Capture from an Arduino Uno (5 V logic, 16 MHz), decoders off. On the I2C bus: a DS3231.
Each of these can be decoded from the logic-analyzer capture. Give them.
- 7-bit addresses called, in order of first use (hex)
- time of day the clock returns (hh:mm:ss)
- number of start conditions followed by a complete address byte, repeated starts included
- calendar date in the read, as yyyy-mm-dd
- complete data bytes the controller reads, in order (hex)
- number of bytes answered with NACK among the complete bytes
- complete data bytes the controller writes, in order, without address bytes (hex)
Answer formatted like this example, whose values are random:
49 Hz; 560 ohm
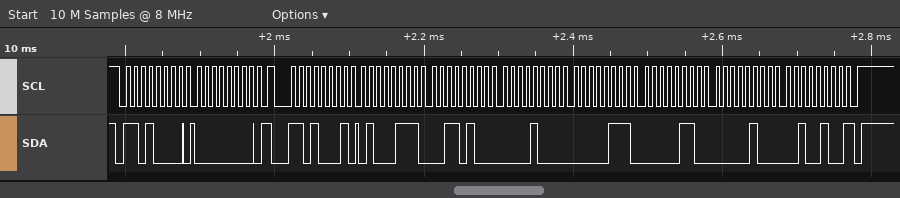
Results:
0x68; 08:34:47; 2; 2024-04-06; 47 34 08 07 06 04 24; 1; 00
